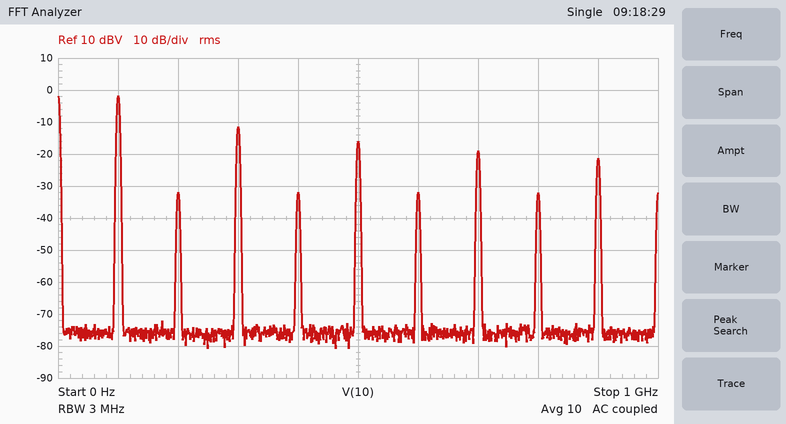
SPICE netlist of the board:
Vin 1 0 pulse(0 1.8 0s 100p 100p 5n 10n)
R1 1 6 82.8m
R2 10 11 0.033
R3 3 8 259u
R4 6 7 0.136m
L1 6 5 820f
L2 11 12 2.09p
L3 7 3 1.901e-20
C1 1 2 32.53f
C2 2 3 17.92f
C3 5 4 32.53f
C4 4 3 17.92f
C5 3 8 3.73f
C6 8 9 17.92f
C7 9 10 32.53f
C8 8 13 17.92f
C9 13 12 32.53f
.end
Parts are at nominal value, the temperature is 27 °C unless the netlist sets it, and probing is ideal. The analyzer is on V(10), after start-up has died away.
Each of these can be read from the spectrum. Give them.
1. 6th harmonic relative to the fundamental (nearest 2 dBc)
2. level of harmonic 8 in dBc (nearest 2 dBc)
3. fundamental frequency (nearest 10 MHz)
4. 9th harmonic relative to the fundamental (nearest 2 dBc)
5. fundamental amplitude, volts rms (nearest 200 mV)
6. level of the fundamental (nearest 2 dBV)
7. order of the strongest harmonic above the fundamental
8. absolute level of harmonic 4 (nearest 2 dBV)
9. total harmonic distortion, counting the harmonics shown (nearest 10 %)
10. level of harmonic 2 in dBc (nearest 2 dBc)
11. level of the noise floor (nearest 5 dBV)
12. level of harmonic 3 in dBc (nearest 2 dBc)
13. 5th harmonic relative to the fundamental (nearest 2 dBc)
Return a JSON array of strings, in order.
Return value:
["-30 dBc", "-30 dBc", "100 MHz", "-20 dBc", "800 mV", "-2 dBV", "3", "-32 dBV", "40 %", "-30 dBc", "-75 dBV", "-10 dBc", "-14 dBc"]
